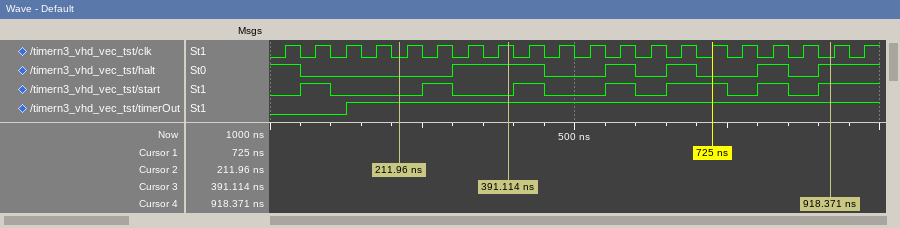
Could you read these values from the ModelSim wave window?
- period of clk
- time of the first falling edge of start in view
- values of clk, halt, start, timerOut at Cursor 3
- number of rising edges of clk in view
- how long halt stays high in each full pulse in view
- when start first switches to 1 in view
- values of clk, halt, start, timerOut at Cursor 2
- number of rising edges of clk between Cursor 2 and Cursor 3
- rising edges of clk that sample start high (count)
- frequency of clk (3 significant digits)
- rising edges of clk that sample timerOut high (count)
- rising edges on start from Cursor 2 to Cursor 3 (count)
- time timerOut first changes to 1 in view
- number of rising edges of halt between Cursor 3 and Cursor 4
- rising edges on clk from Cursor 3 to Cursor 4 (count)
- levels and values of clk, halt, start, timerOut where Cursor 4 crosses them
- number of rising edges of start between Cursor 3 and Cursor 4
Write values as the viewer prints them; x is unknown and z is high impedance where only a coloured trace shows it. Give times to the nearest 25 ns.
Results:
50 ns
100 ns
clk=1, halt=1, start=0, timerOut=1
20
150 ns, 50 ns, 50 ns, 50 ns
50 ns
clk=0, halt=0, start=0, timerOut=1
4
9
20.0 MHz
17
1
125 ns
4
10
clk=0, halt=1, start=1, timerOut=1
5
